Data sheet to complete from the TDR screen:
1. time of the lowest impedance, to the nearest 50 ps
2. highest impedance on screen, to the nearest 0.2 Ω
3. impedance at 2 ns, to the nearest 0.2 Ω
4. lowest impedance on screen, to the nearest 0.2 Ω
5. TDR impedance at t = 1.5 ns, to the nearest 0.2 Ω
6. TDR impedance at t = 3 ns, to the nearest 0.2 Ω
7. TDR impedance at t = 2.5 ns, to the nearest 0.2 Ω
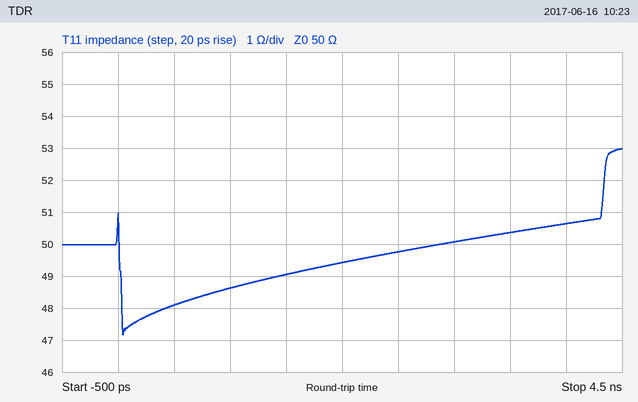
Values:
50 ps
53.0 Ω
49.4 Ω
47.2 Ω
49.0 Ω
50.0 Ω
49.8 Ω
